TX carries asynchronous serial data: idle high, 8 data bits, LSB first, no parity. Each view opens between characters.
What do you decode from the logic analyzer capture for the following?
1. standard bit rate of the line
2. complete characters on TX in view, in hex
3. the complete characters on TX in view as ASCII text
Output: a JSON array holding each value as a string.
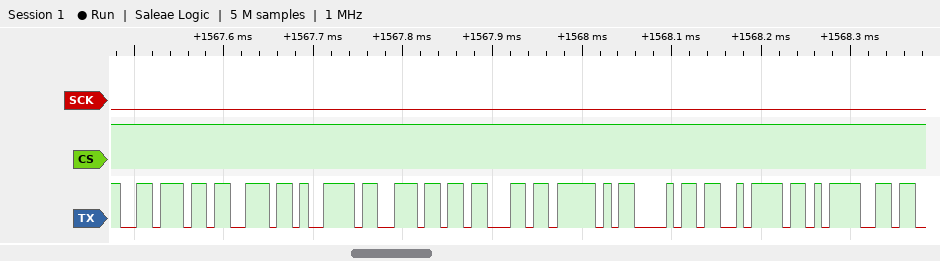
["115200 baud", "76, 73, 79, 6E, 63, 5F, 68, 7A, 3D", "\"vsync_hz=\""]
